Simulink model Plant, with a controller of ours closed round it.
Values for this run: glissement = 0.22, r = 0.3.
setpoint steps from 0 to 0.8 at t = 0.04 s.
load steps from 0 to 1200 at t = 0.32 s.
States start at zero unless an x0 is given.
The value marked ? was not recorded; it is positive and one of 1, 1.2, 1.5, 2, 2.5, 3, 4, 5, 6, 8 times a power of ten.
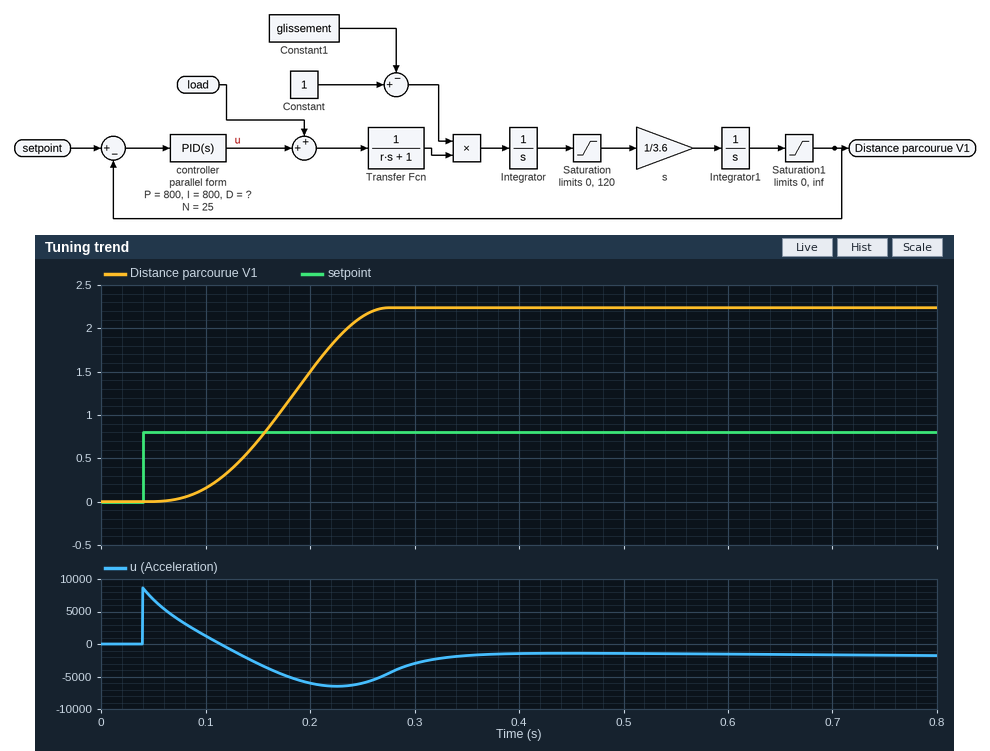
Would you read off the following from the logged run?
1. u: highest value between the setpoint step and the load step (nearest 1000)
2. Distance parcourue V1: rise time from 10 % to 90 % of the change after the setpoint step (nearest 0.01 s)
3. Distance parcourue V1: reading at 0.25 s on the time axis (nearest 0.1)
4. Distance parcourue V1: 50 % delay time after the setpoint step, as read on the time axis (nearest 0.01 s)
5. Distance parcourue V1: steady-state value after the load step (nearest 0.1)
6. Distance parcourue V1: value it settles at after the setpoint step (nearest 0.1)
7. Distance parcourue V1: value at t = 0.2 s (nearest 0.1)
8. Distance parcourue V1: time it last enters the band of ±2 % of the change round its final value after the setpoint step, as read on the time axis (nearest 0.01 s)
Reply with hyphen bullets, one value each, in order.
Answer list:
- 9000
- 0.13 s
- 2.1
- 0.18 s
- 2.2
- 2.2
- 1.5
- 0.26 s
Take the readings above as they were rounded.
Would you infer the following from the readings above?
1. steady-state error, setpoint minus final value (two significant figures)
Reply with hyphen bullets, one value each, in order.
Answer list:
- -1.4
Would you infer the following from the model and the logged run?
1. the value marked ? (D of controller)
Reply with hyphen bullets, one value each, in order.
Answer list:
- 400
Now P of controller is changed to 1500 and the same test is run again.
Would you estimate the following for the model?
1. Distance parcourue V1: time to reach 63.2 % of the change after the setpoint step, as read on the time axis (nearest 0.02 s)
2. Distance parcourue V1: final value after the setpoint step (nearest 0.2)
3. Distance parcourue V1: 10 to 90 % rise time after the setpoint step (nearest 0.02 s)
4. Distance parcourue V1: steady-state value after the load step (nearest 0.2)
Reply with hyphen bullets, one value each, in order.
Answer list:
- 0.20 s
- 2.4
- 0.12 s
- 2.4
